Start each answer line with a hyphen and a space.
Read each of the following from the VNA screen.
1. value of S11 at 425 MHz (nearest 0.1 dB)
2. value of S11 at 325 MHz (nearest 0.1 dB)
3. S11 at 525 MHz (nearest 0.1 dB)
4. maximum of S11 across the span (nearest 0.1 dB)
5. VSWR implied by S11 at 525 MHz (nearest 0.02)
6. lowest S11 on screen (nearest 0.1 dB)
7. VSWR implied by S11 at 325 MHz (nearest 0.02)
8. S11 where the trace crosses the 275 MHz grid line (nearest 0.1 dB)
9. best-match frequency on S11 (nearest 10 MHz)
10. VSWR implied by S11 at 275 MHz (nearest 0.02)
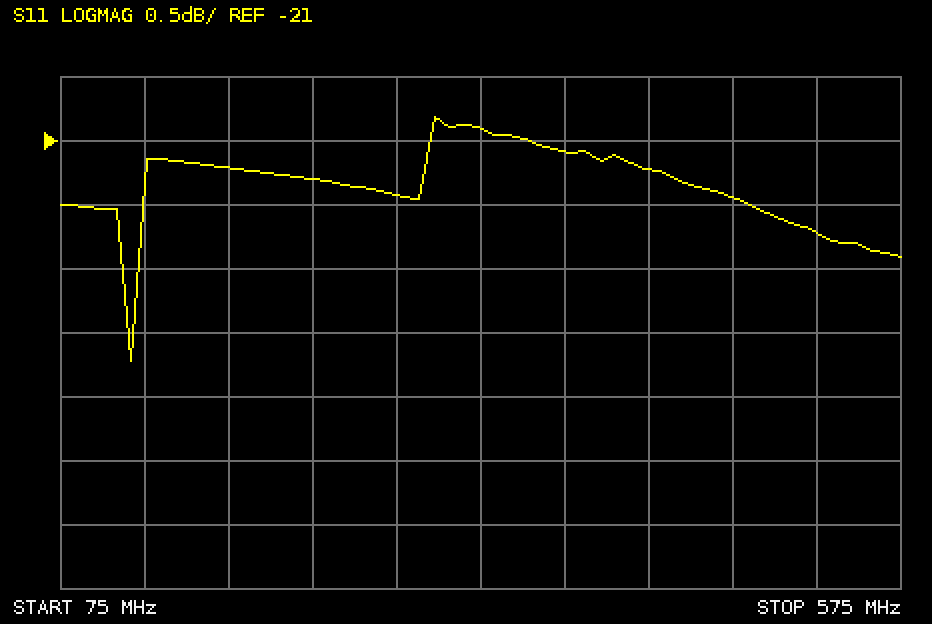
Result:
- -21.2 dB
- -20.9 dB
- -21.7 dB
- -20.8 dB
- 1.18
- -22.7 dB
- 1.20
- -21.4 dB
- 120 MHz
- 1.18
